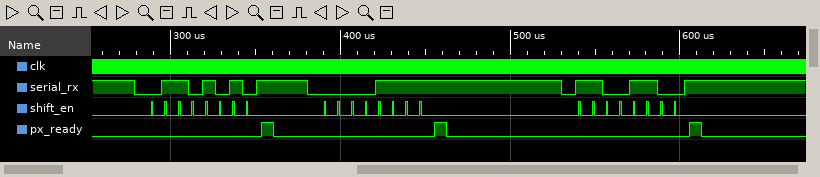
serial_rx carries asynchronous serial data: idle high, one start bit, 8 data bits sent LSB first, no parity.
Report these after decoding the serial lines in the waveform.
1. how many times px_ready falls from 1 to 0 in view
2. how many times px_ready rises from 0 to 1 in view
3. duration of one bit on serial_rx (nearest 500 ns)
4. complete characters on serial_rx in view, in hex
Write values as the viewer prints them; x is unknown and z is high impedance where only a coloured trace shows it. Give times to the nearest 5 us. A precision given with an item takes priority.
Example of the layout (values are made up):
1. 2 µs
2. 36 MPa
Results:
1. 3
2. 3
3. 8000 ns
4. 56, F0, 33
